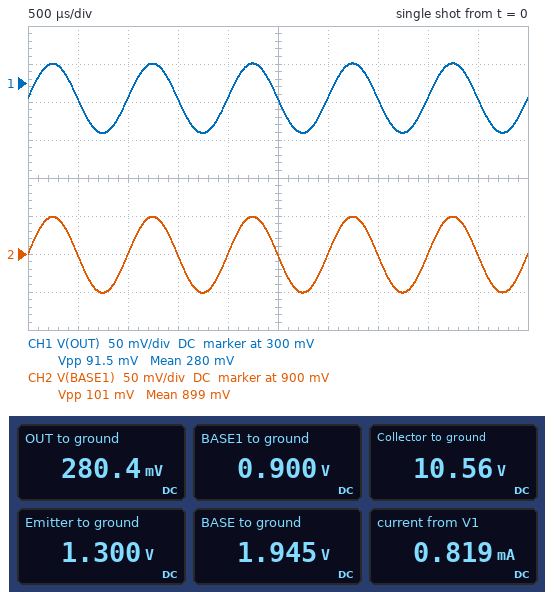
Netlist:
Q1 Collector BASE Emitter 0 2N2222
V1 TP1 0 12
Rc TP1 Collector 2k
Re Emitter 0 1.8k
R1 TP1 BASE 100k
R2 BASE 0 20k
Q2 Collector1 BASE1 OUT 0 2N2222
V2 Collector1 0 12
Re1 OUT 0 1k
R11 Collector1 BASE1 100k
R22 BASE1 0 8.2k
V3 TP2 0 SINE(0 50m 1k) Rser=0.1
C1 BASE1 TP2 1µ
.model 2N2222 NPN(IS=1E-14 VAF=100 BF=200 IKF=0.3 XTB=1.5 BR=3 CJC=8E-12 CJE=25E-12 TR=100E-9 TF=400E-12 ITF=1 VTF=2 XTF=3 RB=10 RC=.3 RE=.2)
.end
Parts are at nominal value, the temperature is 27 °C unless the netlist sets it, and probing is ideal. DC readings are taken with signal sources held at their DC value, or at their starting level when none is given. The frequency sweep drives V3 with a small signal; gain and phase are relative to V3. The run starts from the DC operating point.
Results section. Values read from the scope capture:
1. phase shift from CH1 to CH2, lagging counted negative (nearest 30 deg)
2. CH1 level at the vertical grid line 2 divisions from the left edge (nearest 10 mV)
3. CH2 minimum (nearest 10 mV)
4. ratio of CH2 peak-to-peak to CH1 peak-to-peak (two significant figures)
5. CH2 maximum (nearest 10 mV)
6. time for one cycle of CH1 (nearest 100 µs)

0 deg
280 mV
850 mV
1.1
950 mV
1.0 ms
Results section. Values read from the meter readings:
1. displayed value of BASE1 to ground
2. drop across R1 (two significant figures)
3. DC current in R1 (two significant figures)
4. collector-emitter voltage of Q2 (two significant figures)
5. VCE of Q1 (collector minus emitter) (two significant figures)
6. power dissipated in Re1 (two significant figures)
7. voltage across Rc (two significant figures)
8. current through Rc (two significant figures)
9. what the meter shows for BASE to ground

0.900 V
10 V
100 µA
12 V
9.3 V
79 µW
1.4 V
720 µA
1.945 V
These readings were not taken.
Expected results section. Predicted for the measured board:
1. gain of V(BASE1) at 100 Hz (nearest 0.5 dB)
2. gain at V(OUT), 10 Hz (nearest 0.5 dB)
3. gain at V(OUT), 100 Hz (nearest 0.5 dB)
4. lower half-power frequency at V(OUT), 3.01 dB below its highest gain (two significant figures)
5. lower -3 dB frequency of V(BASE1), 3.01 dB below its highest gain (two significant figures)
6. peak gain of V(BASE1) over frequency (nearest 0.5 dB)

0 dB
-8.5 dB
-1.0 dB
22 Hz
22 Hz
0 dB
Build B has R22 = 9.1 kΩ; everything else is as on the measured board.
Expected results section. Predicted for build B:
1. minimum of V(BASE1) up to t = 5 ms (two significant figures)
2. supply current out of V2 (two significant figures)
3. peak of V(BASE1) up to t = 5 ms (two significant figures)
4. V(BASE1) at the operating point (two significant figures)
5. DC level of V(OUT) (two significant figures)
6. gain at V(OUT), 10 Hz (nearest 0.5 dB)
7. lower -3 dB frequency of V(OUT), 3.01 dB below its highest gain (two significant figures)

940 mV
470 µA
1.0 V
990 mV
360 mV
-7.5 dB
20 Hz
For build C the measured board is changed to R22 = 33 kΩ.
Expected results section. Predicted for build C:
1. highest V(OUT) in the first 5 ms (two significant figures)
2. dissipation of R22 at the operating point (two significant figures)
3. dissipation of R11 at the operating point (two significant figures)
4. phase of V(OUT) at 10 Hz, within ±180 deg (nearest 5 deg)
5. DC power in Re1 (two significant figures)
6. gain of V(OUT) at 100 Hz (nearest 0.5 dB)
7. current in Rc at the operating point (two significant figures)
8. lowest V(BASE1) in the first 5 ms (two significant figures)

2.1 V
230 µW
860 µW
35 deg
4.3 mW
0 dB
720 µA
2.7 V
